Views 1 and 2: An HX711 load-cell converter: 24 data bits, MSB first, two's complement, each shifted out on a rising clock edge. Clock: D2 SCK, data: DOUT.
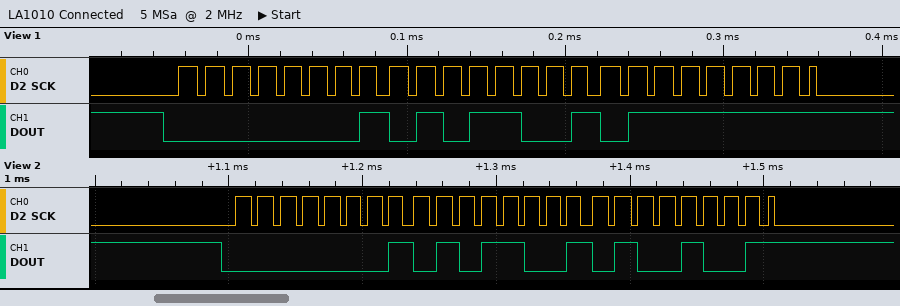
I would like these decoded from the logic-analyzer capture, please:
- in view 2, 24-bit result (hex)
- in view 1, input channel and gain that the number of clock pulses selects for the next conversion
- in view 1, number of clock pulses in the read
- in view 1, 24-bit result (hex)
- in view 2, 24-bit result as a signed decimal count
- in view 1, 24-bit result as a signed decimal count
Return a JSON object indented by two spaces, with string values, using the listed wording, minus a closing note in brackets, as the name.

{
  "in view 2, 24-bit result": "0x015949",
  "in view 1, input channel and gain that the number of clock pulses selects for the next conversion": "channel A, gain 128",
  "in view 1, number of clock pulses in the read": "25",
  "in view 1, 24-bit result": "0x01597F",
  "in view 2, 24-bit result as a signed decimal count": "88393",
  "in view 1, 24-bit result as a signed decimal count": "88447"
}
